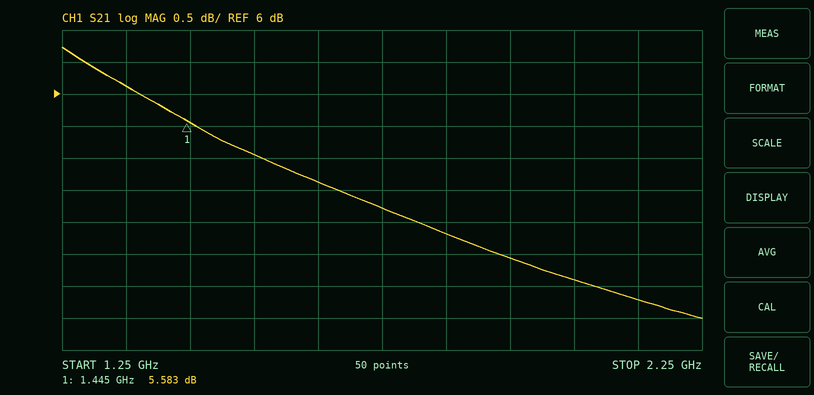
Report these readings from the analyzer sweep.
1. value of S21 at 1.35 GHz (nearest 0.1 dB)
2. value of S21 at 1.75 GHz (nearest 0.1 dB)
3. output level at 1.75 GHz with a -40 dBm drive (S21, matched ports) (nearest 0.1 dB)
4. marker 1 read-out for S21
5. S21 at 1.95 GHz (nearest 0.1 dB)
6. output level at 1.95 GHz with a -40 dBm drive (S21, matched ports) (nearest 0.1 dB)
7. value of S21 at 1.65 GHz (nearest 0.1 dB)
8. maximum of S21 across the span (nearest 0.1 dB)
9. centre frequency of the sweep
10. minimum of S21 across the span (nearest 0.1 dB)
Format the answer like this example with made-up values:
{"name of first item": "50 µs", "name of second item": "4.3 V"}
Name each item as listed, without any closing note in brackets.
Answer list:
{"value of S21 at 1.35 GHz": "6.1 dB", "value of S21 at 1.75 GHz": "4.2 dB", "output level at 1.75 GHz with a -40 dBm drive (S21, matched ports)": "-35.8 dBm", "marker 1 read-out for S21": "5.583 dB", "S21 at 1.95 GHz": "3.4 dB", "output level at 1.95 GHz with a -40 dBm drive (S21, matched ports)": "-36.6 dBm", "value of S21 at 1.65 GHz": "4.6 dB", "maximum of S21 across the span": "6.7 dB", "centre frequency of the sweep": "1.75 GHz", "minimum of S21 across the span": "2.5 dB"}
